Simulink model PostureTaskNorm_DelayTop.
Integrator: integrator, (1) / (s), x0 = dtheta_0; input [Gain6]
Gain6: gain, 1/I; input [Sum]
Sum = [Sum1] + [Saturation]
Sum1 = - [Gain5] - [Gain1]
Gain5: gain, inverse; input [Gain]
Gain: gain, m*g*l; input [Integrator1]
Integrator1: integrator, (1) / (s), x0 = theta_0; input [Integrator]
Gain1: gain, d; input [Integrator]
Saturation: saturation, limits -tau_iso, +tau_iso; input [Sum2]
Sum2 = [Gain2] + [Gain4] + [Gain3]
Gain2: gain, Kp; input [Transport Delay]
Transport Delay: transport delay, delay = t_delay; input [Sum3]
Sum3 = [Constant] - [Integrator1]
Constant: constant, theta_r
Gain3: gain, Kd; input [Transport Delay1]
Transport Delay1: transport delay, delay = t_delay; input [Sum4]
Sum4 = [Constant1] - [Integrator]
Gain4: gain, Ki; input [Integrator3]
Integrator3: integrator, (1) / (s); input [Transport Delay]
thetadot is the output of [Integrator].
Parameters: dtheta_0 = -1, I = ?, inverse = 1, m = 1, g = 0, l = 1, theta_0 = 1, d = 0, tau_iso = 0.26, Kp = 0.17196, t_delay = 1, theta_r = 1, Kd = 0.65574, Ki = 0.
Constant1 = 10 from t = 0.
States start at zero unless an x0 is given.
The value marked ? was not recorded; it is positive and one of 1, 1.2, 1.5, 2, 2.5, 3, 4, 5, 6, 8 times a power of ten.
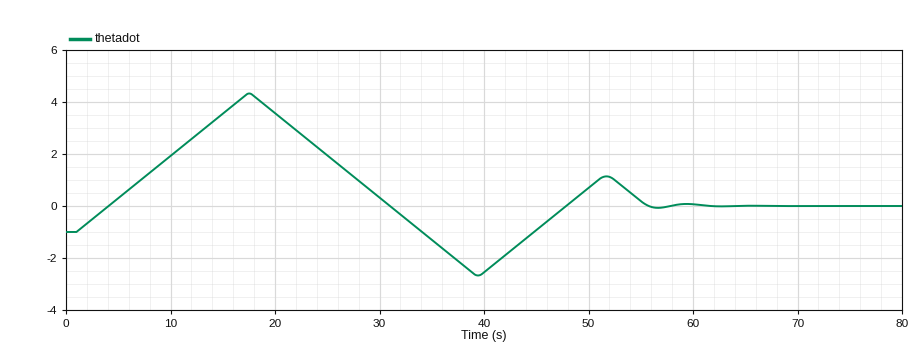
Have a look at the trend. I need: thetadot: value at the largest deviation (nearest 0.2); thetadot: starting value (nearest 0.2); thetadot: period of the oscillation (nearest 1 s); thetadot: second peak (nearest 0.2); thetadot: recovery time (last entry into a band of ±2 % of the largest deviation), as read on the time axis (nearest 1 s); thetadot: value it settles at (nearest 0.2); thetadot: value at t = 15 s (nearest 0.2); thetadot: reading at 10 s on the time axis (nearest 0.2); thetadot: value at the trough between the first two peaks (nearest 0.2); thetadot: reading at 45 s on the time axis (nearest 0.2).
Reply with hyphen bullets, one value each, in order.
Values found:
- 4.4
- -1.0
- 34 s
- 1.2
- 55 s
- 0.0
- 3.6
- 2.0
- -2.6
- -1.0
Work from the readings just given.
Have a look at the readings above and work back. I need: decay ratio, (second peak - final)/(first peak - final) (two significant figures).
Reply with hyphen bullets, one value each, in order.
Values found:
- 0.27
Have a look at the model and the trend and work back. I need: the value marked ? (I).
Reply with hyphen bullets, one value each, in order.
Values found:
- 0.8
